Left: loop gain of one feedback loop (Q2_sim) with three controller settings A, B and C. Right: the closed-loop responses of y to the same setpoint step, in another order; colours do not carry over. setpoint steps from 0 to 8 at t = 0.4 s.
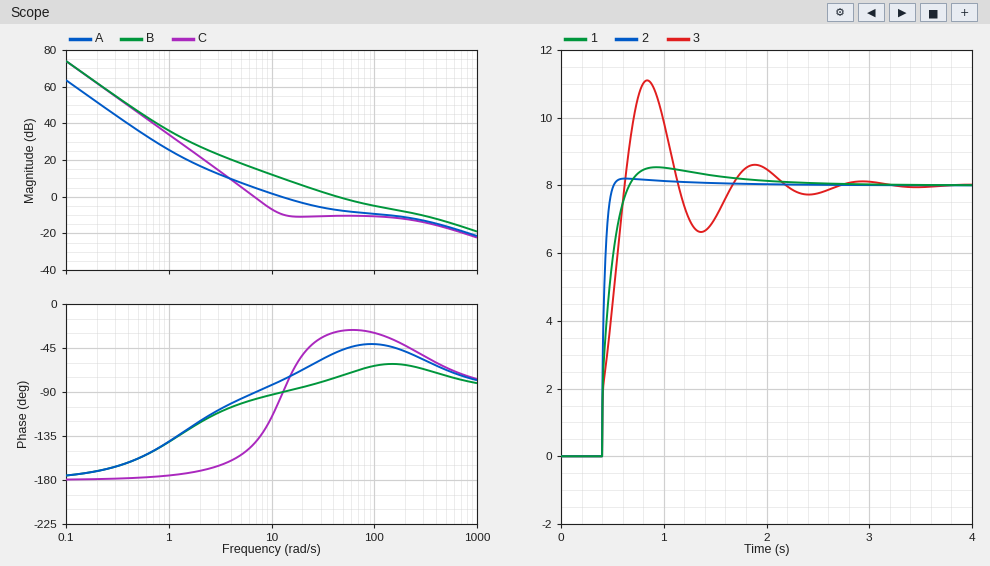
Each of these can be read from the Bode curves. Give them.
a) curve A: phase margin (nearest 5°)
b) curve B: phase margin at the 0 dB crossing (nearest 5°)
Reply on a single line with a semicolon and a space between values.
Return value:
100°; 105°
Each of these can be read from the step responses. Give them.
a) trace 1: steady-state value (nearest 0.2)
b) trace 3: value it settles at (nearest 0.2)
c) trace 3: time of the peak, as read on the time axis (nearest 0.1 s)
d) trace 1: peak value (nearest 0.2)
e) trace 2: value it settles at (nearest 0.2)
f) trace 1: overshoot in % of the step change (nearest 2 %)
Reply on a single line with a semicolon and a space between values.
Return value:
8.0; 8.0; 0.8 s; 8.6; 8.0; 6 %
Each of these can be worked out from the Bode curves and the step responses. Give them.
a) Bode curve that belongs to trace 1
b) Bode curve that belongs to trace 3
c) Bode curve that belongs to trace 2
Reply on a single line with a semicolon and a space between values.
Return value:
A; C; B
